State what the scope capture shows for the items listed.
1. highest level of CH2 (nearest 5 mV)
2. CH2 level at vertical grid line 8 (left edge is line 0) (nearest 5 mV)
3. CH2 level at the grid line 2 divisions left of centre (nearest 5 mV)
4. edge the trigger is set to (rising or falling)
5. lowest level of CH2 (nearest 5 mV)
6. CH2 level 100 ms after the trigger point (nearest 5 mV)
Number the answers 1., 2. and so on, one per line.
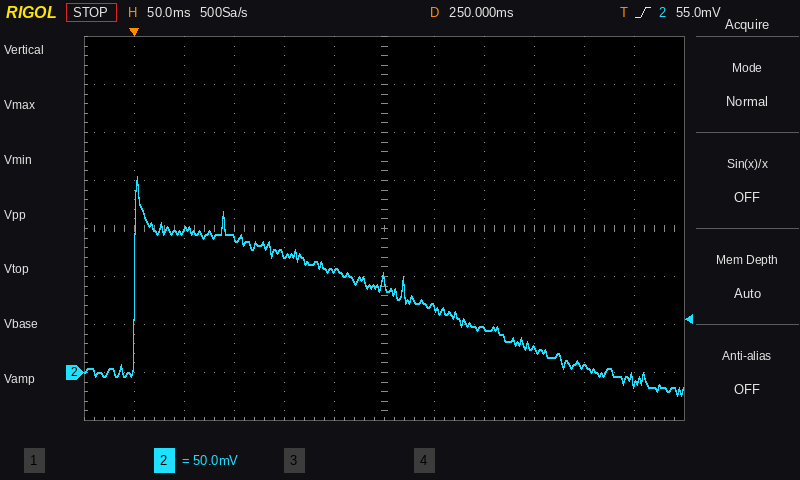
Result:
1. 205 mV
2. 45 mV
3. 125 mV
4. rising
5. -25 mV
6. 140 mV
